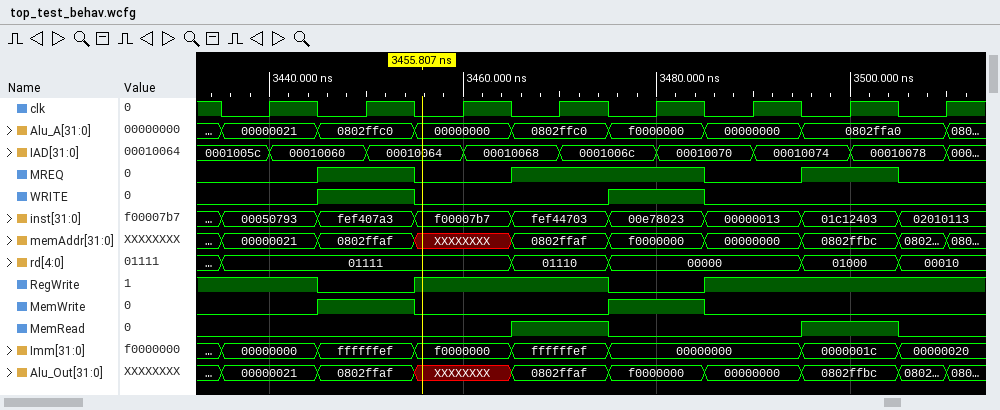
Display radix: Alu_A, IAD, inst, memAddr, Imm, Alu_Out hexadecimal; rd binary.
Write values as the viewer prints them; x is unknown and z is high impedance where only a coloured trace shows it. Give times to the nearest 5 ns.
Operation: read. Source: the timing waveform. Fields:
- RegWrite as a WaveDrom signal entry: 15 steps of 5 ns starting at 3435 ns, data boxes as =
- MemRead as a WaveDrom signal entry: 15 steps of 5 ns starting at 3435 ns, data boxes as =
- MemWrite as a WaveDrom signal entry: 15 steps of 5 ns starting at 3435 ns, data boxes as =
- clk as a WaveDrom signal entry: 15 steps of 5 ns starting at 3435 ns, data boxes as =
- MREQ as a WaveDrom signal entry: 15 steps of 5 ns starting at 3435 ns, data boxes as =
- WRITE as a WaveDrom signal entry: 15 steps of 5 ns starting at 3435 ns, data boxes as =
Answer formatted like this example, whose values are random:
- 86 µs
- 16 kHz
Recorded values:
- {name: 'RegWrite', wave: '1.0.1...0.1....'}
- {name: 'MemRead', wave: '0.....1.0...1.0'}
- {name: 'MemWrite', wave: '0.1.0...1.0....'}
- {name: 'clk', wave: '010101010101010'}
- {name: 'MREQ', wave: '0.1.0.1...0.1.0'}
- {name: 'WRITE', wave: '0.1.0...1.0....'}
